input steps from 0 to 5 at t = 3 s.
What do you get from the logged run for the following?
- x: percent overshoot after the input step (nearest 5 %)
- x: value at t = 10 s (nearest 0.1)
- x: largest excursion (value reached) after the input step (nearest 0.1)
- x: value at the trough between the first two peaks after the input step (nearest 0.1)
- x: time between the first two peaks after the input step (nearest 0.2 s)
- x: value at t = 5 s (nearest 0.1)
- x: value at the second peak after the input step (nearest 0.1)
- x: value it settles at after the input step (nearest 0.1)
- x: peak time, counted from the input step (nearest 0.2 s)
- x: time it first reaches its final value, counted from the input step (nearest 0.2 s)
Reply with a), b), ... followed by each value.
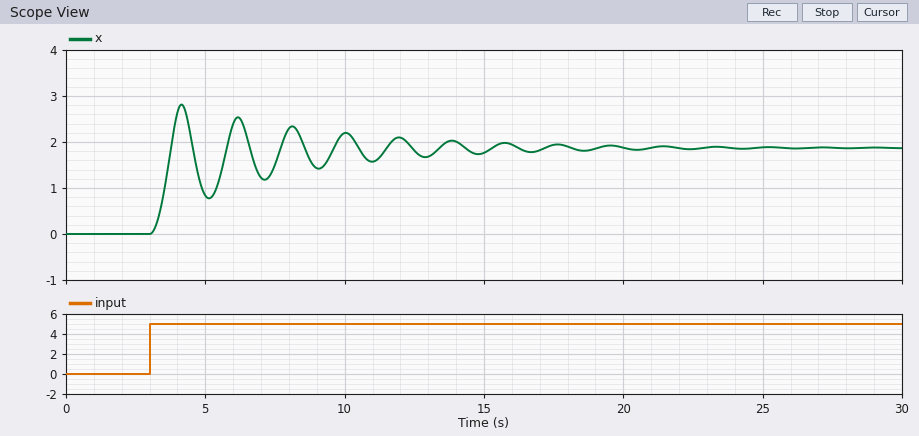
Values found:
a) 50 %
b) 2.2
c) 2.8
d) 0.8
e) 2.0 s
f) 0.8
g) 2.5
h) 1.9
i) 1.2 s
j) 0.8 s
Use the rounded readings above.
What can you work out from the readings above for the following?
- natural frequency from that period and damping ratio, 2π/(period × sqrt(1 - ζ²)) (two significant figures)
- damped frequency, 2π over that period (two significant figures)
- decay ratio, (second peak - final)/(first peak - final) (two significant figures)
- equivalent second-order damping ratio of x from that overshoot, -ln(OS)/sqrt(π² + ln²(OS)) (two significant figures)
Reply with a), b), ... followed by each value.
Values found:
a) 3.2 rad/s
b) 3.1 rad/s
c) 0.67
d) 0.22
